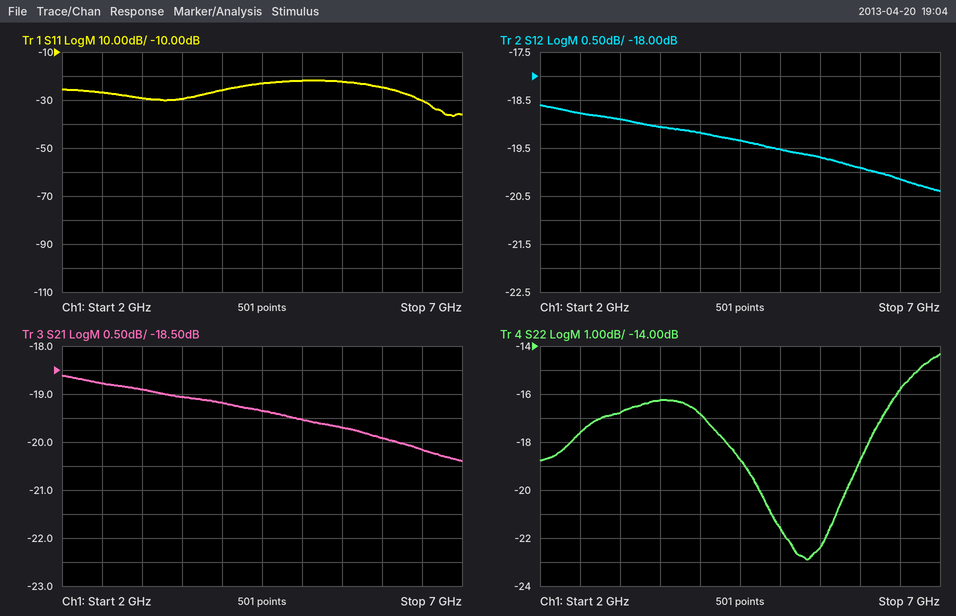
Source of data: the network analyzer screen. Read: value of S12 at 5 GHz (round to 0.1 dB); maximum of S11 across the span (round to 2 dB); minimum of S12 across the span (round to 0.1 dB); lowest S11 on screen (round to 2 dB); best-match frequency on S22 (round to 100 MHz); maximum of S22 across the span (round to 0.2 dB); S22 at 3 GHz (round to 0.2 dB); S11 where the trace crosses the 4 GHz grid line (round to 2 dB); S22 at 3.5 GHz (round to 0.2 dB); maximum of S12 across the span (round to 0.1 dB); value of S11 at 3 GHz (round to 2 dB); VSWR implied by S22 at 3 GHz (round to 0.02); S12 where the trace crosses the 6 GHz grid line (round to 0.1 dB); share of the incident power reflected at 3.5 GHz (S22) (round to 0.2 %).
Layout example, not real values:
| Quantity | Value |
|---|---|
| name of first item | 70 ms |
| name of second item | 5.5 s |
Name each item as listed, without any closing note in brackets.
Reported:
| Quantity | Value |
|---|---|
| value of S12 at 5 GHz | -19.5 dB |
| maximum of S11 across the span | -22 dB |
| minimum of S12 across the span | -20.4 dB |
| lowest S11 on screen | -36 dB |
| best-match frequency on S22 | 5.3 GHz |
| maximum of S22 across the span | -14.4 dB |
| S22 at 3 GHz | -16.8 dB |
| S11 where the trace crosses the 4 GHz grid line | -26 dB |
| S22 at 3.5 GHz | -16.2 dB |
| maximum of S12 across the span | -18.6 dB |
| value of S11 at 3 GHz | -30 dB |
| VSWR implied by S22 at 3 GHz | 1.34 |
| S12 where the trace crosses the 6 GHz grid line | -19.9 dB |
| share of the incident power reflected at 3.5 GHz (S22) | 2.4 % |
